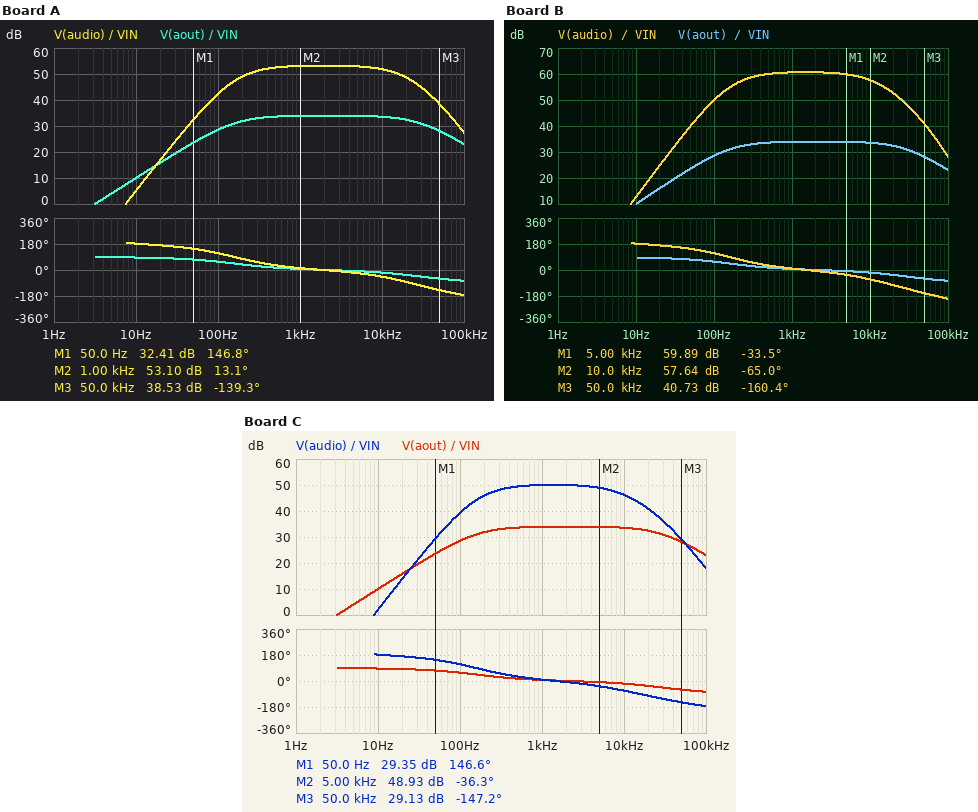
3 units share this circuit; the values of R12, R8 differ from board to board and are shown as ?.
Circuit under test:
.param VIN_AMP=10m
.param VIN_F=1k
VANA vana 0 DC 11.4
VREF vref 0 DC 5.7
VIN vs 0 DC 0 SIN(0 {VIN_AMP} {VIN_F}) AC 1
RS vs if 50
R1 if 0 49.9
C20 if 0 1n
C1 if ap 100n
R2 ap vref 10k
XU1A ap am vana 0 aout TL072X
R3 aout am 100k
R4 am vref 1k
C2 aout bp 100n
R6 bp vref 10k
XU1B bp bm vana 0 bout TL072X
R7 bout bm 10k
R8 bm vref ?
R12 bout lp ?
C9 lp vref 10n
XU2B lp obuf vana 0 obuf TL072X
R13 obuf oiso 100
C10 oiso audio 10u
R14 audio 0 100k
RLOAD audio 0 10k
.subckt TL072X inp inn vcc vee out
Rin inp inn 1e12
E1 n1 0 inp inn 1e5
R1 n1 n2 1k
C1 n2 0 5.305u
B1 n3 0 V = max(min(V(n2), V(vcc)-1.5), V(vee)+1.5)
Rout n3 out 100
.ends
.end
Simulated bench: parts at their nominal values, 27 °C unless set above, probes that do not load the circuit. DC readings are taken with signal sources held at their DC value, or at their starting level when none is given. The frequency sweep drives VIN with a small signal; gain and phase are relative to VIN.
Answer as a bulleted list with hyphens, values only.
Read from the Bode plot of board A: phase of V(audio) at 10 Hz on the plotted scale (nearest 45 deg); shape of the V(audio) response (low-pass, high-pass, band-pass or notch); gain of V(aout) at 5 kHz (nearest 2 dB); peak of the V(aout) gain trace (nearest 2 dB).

- 180 deg
- band-pass
- 34 dB
- 34 dB
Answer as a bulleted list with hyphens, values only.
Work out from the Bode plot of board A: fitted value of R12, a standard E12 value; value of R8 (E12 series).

- 820 Ω
- 1.2 kΩ
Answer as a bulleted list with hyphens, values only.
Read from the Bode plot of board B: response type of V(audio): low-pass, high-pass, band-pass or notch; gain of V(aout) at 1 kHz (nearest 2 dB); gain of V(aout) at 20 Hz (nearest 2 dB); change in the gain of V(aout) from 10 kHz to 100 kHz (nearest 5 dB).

- band-pass
- 34 dB
- 16 dB
- -10 dB
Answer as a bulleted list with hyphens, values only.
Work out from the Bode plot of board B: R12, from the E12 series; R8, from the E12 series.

- 1.5 kΩ
- 470 Ω
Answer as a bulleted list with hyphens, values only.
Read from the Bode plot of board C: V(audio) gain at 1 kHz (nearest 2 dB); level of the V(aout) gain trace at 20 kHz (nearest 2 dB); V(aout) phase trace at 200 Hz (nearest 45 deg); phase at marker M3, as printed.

- 50 dB
- 32 dB
- 45 deg
- -147.2 deg
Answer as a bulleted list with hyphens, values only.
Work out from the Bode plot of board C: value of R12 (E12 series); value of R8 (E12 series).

- 1.8 kΩ
- 1.8 kΩ
